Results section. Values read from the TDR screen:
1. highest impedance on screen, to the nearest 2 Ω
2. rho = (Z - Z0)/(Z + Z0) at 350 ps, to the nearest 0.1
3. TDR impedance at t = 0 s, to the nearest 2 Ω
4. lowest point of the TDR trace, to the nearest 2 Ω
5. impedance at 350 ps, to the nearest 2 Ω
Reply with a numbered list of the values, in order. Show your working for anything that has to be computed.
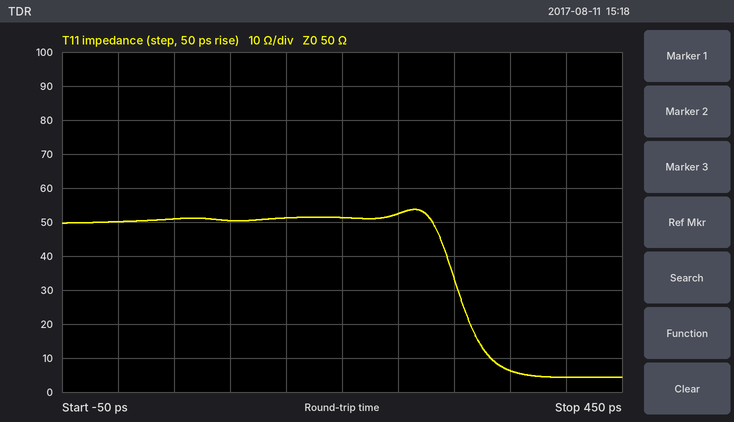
1. 54 Ω
2. (6 − 50)/(6 + 50) ≈ -0.8
3. 50 Ω
4. 4 Ω
5. 6 Ω
